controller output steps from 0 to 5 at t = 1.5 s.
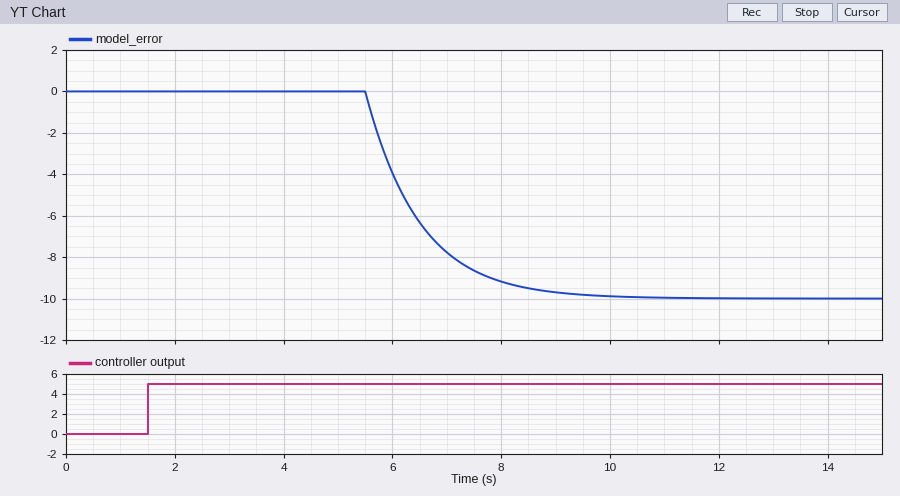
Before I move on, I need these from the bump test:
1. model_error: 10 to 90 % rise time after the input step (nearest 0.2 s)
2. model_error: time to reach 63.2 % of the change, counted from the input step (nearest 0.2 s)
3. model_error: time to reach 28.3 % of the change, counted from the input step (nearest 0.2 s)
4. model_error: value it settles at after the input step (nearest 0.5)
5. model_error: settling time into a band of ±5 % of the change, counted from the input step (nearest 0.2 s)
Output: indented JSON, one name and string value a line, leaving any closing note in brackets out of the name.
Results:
{
  "model_error: 10 to 90 % rise time after the input step": "2.2 s",
  "model_error: time to reach 63.2 % of the change, counted from the input step": "5.0 s",
  "model_error: time to reach 28.3 % of the change, counted from the input step": "4.4 s",
  "model_error: value it settles at after the input step": "-10.0",
  "model_error: settling time into a band of ±5 % of the change, counted from the input step": "7.0 s"
}
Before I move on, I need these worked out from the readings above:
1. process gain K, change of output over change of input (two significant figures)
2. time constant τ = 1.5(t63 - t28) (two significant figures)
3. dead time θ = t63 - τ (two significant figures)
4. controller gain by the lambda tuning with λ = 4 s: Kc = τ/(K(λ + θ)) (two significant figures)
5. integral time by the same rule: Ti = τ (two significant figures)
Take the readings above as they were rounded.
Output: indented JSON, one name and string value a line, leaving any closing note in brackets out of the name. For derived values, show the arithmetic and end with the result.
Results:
{
  "process gain K, change of output over change of input": "(-10 - 0) / 5 = -2.0",
  "time constant τ = 1.5(t63 - t28)": "1.5 × (5 - 4.4) = 0.90 s",
  "dead time θ = t63 - τ": "5 - 0.9 = 4.1 s",
  "controller gain by the lambda tuning with λ = 4 s: Kc = τ/(K(λ + θ))": "0.9 / (-2 × (4 + 4.1)) = -0.056",
  "integral time by the same rule: Ti = τ": "0.90 s"
}
